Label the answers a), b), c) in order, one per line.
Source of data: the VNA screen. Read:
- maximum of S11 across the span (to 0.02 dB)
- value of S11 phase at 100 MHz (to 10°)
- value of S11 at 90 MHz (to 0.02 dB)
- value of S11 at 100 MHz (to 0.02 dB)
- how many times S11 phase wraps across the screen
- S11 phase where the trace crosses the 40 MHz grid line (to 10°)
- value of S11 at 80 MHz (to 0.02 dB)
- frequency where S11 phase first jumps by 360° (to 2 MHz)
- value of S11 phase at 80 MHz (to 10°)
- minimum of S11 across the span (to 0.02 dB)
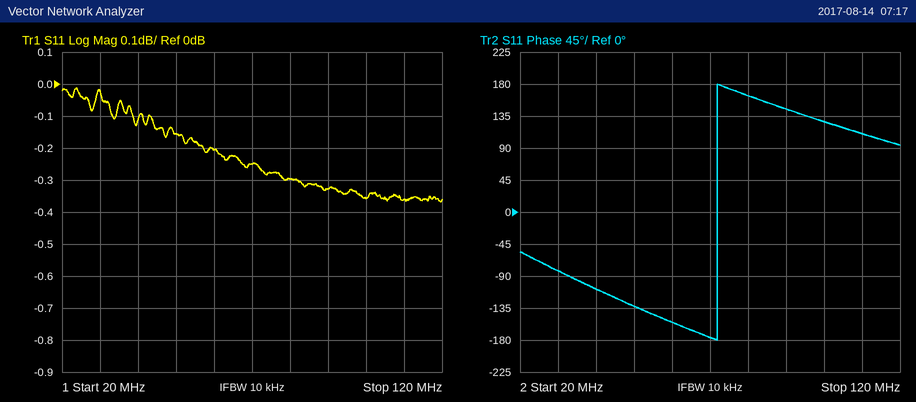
a) -0.02 dB
b) 130°
c) -0.32 dB
d) -0.36 dB
e) 1
f) -110°
g) -0.30 dB
h) 72 MHz
i) 160°
j) -0.36 dB
